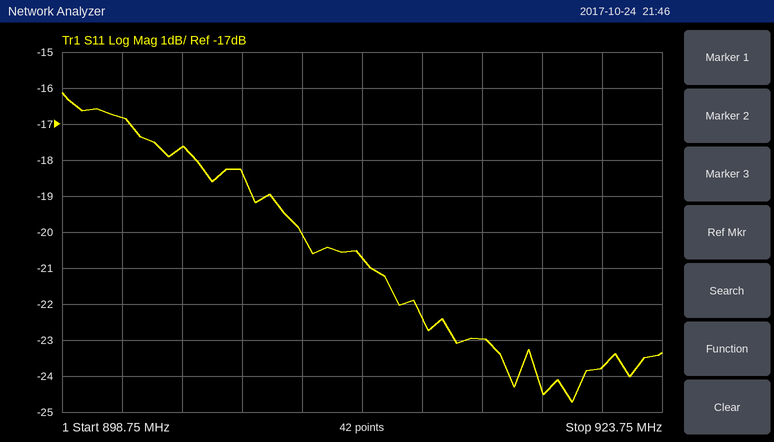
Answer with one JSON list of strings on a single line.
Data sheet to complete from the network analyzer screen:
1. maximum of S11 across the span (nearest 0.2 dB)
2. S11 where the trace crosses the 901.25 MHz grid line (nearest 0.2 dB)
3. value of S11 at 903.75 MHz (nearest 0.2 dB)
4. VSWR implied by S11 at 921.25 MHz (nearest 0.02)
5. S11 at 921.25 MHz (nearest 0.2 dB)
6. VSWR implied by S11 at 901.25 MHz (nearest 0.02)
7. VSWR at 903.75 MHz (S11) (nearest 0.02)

["-16.2 dB", "-16.8 dB", "-17.6 dB", "1.14", "-23.8 dB", "1.34", "1.30"]
